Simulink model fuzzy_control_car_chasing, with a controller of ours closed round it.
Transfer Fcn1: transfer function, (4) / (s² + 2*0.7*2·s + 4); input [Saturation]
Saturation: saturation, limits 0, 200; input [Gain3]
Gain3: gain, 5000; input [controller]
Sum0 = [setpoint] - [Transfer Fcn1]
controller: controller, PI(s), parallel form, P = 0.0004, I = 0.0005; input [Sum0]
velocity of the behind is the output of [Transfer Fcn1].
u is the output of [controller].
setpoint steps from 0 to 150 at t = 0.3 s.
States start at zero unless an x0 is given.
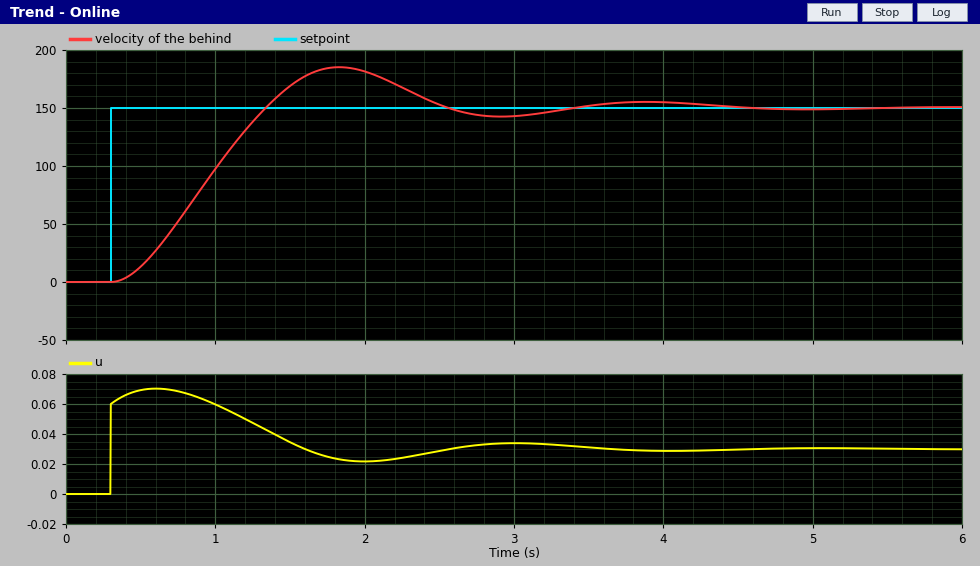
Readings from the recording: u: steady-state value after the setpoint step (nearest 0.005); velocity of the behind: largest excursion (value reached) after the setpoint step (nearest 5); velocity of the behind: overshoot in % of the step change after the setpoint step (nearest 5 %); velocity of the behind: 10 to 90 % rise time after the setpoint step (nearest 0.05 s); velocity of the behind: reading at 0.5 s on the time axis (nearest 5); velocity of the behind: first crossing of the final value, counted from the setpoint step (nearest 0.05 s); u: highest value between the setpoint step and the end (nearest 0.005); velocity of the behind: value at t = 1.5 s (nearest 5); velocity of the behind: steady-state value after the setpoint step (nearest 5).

0.030
185
25 %
0.70 s
15
1.05 s
0.070
170
150
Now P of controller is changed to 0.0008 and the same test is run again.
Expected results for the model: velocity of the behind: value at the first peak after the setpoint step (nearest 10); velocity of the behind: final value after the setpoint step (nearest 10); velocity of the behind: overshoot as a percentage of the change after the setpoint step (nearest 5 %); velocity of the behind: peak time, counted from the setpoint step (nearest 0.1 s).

180
150
20 %
1.4 s
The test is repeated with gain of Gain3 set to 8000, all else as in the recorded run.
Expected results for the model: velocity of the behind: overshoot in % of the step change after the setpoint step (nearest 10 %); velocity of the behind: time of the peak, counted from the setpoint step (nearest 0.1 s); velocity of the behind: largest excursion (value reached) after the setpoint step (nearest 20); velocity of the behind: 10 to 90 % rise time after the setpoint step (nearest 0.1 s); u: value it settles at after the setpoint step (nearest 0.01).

30 %
1.7 s
200
0.7 s
0.02
